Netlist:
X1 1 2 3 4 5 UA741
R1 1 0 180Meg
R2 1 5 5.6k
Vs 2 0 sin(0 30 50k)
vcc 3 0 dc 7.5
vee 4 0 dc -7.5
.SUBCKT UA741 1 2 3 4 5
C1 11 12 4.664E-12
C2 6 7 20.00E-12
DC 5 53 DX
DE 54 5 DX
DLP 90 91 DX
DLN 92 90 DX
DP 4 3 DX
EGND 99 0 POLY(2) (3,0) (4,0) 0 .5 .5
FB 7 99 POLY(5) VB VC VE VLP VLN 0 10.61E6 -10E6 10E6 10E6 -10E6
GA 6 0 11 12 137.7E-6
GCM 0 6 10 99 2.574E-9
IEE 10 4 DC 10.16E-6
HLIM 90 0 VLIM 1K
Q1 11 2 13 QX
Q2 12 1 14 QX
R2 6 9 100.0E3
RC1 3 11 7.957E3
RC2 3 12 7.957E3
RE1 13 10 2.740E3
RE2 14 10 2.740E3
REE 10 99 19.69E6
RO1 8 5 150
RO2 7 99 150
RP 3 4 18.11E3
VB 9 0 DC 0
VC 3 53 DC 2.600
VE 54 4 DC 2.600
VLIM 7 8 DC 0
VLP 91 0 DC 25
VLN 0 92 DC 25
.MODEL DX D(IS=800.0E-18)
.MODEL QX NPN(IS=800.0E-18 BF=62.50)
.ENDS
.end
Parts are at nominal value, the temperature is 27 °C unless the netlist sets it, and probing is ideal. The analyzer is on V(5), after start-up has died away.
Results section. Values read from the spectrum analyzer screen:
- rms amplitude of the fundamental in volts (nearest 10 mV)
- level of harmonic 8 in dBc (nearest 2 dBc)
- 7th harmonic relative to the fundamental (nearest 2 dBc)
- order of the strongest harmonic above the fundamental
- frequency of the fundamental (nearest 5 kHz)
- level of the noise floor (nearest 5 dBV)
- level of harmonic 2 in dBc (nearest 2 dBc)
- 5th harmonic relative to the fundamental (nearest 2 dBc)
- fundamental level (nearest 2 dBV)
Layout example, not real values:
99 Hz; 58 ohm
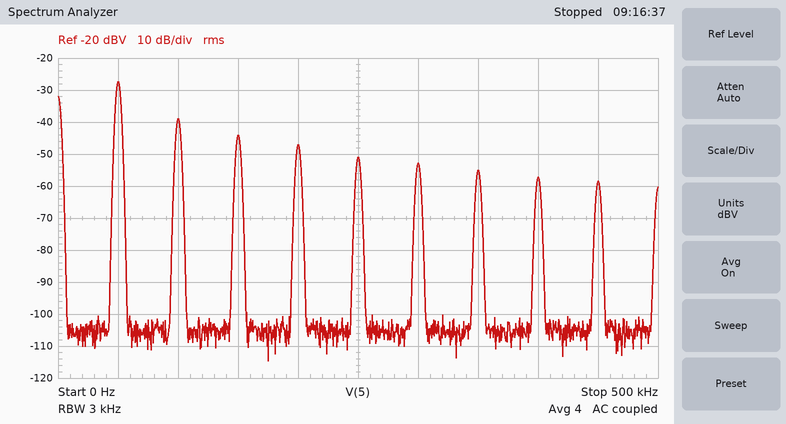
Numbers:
40 mV; -30 dBc; -28 dBc; 2; 50 kHz; -105 dBV; -12 dBc; -24 dBc; -28 dBV
